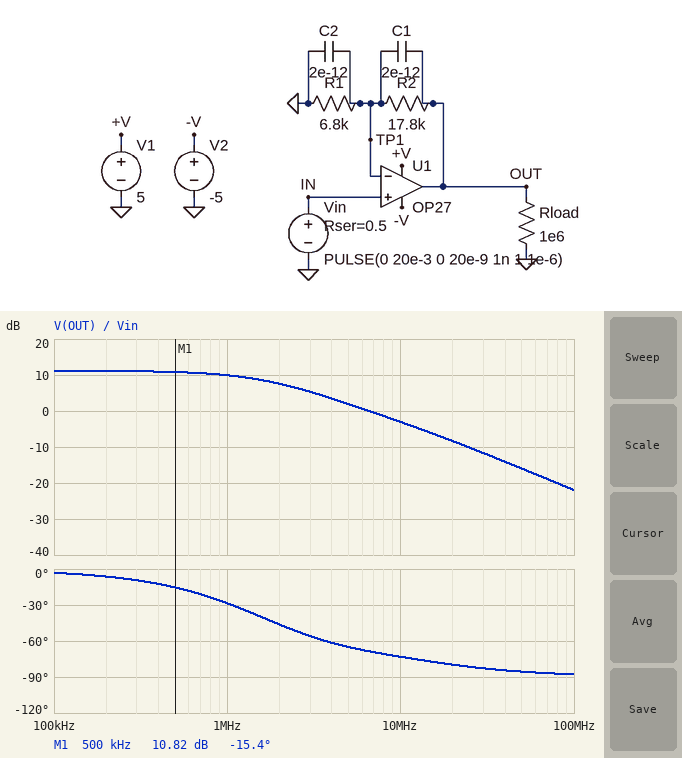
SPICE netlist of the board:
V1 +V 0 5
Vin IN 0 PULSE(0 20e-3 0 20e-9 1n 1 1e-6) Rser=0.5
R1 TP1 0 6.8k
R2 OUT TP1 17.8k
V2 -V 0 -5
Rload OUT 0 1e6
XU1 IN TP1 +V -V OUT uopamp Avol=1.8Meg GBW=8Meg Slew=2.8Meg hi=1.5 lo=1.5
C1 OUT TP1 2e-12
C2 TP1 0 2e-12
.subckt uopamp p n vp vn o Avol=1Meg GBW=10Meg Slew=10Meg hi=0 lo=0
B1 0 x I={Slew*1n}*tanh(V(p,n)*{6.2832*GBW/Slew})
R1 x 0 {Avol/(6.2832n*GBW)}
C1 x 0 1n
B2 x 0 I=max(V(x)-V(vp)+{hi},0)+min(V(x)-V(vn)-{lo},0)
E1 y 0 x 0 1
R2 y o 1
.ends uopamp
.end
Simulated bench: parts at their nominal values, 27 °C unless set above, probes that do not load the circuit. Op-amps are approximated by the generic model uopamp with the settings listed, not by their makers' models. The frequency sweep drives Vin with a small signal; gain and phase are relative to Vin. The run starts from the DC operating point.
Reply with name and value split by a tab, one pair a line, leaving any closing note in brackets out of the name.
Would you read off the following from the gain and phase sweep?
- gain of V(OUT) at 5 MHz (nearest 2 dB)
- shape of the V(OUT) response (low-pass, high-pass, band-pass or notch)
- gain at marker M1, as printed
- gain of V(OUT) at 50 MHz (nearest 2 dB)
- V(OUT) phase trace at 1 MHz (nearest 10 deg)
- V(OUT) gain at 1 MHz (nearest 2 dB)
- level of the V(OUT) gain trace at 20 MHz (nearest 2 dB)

gain of V(OUT) at 5 MHz	2 dB
shape of the V(OUT) response	low-pass
gain at marker M1, as printed	10.82 dB
gain of V(OUT) at 50 MHz	-16 dB
V(OUT) phase trace at 1 MHz	-30 deg
V(OUT) gain at 1 MHz	10 dB
level of the V(OUT) gain trace at 20 MHz	-8 dB
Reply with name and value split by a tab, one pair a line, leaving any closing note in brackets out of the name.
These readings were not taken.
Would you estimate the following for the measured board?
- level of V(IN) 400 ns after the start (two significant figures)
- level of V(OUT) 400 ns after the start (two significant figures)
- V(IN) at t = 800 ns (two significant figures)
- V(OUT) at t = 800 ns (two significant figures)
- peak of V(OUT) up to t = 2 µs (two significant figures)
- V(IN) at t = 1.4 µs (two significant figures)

level of V(IN) 400 ns after the start	20 mV
level of V(OUT) 400 ns after the start	71 mV
V(IN) at t = 800 ns	20 mV
V(OUT) at t = 800 ns	72 mV
peak of V(OUT) up to t = 2 µs	72 mV
V(IN) at t = 1.4 µs	20 mV
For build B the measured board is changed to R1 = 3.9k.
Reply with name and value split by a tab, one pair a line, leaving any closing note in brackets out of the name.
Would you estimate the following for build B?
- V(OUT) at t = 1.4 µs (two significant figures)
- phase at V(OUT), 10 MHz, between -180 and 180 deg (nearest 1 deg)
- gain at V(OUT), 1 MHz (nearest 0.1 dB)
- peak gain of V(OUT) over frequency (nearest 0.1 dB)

V(OUT) at t = 1.4 µs	110 mV
phase at V(OUT), 10 MHz, between -180 and 180 deg	-78 deg
gain at V(OUT), 1 MHz	12.5 dB
peak gain of V(OUT) over frequency	14.9 dB
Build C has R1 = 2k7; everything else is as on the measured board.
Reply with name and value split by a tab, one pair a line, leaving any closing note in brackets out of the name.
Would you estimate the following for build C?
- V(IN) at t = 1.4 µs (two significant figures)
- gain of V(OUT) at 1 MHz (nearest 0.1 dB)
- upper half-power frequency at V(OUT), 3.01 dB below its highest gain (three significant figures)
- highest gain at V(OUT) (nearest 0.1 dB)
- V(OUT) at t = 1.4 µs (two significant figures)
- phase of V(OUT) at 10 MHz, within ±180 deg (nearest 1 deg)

V(IN) at t = 1.4 µs	20 mV
gain of V(OUT) at 1 MHz	14.1 dB
upper half-power frequency at V(OUT), 3.01 dB below its highest gain	891 kHz
highest gain at V(OUT)	17.6 dB
V(OUT) at t = 1.4 µs	150 mV
phase of V(OUT) at 10 MHz, within ±180 deg	-81 deg
